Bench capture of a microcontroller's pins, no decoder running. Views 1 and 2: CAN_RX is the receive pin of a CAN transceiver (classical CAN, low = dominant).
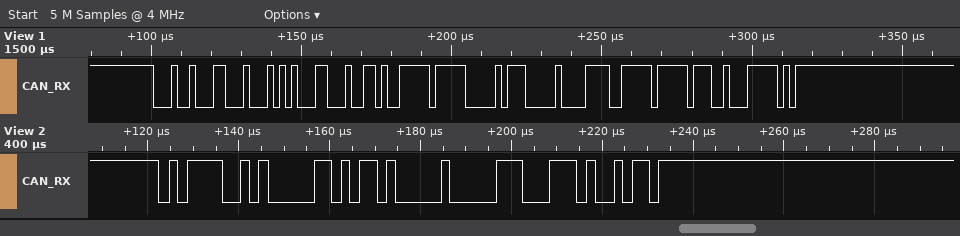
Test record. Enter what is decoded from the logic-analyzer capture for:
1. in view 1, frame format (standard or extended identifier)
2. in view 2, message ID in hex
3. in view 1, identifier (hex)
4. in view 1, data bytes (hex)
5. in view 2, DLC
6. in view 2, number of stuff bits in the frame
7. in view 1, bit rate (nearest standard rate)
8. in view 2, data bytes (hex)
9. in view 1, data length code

standard
0x5E5
0x123
A8 C4 D3 FF 07 00 79 FF
2
3
500 kbit/s
B4 00
8
